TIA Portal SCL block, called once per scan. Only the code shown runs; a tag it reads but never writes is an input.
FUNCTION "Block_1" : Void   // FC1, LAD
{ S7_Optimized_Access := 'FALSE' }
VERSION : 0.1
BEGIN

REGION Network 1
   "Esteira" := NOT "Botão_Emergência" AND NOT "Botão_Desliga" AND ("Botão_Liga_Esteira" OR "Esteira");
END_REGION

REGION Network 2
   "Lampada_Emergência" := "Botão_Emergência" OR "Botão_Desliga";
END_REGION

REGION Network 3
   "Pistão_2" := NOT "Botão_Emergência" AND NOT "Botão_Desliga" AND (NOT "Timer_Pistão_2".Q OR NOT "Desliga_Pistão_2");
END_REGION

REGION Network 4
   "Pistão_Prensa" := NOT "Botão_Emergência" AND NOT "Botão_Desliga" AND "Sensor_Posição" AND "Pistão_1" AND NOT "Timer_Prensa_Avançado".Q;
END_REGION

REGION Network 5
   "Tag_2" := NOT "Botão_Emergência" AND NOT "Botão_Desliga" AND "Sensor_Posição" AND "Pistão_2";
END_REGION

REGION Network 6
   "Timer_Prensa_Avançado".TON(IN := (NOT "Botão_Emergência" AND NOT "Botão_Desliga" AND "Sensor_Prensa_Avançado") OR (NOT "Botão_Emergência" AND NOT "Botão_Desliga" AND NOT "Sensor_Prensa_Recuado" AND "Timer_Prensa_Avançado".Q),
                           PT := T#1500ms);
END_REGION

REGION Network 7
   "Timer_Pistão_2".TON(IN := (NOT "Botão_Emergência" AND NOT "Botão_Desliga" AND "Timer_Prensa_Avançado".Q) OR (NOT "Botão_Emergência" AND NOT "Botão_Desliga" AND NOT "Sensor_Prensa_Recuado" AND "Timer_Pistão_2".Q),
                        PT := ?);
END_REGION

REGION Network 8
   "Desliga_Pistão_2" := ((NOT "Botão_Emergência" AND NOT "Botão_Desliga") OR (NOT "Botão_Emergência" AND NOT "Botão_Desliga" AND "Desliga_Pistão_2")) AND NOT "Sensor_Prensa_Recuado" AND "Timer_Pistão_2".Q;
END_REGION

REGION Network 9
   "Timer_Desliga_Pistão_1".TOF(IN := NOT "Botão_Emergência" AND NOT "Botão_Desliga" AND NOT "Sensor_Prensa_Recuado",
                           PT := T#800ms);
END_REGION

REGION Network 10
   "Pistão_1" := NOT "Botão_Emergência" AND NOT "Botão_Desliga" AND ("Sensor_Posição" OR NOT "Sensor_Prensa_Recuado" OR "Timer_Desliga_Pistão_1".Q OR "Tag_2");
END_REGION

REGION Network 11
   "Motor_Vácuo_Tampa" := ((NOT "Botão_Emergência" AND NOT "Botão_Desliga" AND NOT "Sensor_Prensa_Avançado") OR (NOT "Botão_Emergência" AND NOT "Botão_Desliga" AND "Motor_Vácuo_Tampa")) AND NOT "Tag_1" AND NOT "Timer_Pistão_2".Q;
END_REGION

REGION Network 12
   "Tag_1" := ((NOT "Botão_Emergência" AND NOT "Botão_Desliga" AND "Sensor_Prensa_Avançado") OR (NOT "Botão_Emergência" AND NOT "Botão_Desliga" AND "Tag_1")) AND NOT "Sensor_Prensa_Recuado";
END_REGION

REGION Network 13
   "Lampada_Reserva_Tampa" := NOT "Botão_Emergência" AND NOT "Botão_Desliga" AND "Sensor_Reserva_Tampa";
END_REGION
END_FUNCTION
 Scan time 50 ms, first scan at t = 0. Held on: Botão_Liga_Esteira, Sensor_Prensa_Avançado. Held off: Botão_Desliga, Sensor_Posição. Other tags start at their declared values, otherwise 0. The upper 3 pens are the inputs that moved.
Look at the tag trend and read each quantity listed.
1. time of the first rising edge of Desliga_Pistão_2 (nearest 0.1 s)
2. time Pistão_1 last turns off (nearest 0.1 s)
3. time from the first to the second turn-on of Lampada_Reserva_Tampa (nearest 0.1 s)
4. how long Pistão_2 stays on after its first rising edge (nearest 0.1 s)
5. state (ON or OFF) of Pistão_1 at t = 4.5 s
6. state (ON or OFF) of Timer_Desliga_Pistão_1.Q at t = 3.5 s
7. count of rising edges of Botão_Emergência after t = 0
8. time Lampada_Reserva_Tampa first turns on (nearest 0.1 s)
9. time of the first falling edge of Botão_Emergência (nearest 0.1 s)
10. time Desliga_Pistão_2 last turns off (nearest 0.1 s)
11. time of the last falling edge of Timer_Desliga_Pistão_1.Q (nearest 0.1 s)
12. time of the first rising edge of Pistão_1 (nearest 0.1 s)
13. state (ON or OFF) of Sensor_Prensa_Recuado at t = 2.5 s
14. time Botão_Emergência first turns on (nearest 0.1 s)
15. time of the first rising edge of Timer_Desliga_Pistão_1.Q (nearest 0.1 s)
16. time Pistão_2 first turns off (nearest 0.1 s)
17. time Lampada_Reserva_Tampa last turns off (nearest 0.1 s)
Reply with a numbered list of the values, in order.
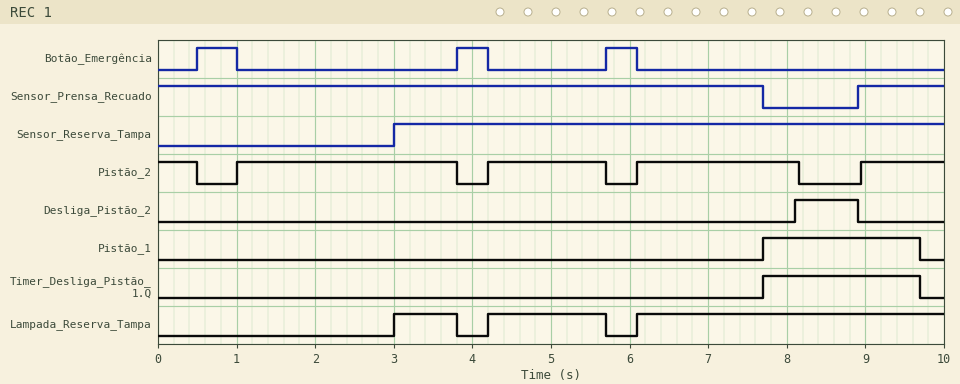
1. 8.1 s
2. 9.7 s
3. 1.2 s
4. 2.8 s
5. OFF
6. OFF
7. 3
8. 3.0 s
9. 1.0 s
10. 8.9 s
11. 9.7 s
12. 7.7 s
13. ON
14. 0.5 s
15. 7.7 s
16. 0.5 s
17. 5.7 s
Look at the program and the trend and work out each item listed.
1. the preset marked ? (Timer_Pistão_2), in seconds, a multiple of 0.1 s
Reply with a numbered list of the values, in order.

1. 0.5 s
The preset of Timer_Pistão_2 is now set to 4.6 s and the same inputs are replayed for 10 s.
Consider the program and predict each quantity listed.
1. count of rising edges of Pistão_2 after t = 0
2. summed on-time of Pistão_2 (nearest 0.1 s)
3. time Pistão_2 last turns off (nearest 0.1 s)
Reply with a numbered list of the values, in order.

1. 3
2. 8.7 s
3. 5.7 s
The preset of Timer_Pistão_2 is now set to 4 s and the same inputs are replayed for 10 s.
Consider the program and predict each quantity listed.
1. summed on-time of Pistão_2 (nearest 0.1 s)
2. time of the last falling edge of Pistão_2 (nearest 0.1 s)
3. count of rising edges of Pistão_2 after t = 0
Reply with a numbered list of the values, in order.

1. 8.7 s
2. 5.7 s
3. 3
